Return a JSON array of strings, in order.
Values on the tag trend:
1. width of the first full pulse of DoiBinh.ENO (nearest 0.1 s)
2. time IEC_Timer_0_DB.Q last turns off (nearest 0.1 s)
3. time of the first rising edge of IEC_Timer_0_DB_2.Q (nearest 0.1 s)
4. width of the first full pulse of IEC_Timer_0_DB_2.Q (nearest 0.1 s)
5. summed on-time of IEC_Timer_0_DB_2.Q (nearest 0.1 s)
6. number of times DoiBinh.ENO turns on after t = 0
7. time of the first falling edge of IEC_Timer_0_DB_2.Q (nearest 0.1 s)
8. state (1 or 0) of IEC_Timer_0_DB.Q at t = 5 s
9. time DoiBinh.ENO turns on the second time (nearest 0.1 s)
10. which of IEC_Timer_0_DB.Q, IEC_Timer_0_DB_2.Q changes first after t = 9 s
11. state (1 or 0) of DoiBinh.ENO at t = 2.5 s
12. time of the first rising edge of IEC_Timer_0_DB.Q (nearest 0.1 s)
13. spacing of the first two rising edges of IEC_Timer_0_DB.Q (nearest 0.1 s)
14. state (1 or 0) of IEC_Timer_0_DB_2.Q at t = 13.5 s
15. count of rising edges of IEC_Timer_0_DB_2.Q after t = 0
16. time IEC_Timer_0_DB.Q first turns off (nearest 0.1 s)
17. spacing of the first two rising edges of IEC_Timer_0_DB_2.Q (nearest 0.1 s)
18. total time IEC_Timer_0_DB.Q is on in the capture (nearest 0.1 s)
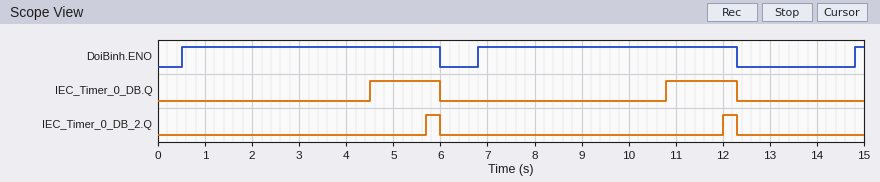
["5.5 s", "12.3 s", "5.7 s", "0.3 s", "0.6 s", "3", "6.0 s", "1", "6.8 s", "IEC_Timer_0_DB.Q", "1", "4.5 s", "6.3 s", "0", "2", "6.0 s", "6.3 s", "3.0 s"]
